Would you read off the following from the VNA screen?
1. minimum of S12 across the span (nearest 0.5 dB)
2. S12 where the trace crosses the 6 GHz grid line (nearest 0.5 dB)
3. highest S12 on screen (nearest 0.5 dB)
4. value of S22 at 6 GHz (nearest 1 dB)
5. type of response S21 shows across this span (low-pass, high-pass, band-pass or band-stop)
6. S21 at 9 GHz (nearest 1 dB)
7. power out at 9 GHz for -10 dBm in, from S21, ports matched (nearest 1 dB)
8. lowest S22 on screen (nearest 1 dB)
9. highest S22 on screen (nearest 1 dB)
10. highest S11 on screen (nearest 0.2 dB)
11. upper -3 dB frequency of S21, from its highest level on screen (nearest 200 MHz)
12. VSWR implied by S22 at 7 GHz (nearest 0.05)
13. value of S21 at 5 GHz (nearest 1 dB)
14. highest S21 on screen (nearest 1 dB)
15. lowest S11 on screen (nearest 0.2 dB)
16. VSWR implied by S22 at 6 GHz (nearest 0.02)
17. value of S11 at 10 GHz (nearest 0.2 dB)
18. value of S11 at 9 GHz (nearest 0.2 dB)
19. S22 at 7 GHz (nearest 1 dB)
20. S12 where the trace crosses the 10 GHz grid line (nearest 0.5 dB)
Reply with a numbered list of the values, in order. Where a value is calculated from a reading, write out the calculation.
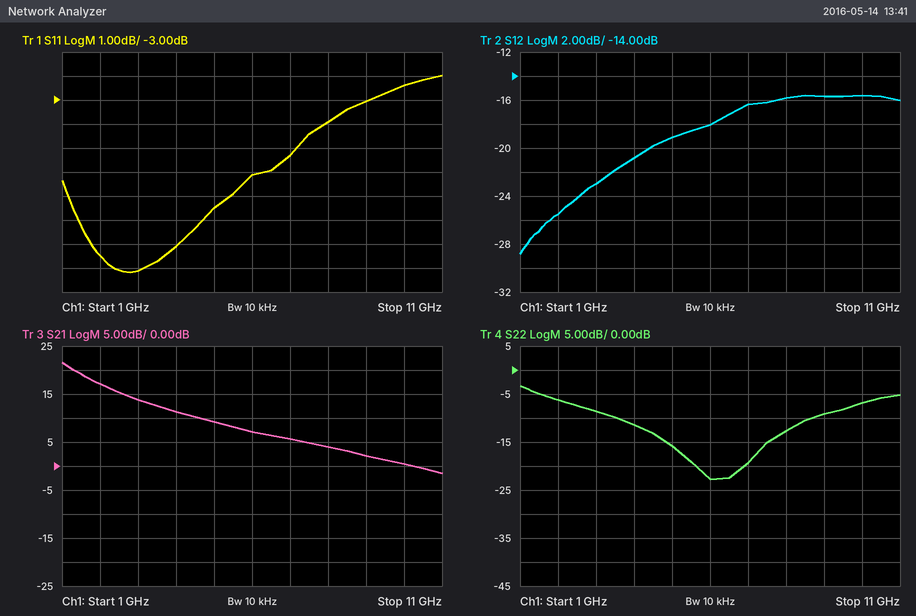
1. -29.0 dB
2. -18.0 dB
3. -15.5 dB
4. -23 dB
5. low-pass
6. 2 dB
7. -10 dBm + (2 dB) = -8 dBm
8. -23 dB
9. -3 dB
10. -2.0 dB
11. 1.6 GHz
12. |Γ| = 10^(-19/20) = 0.1122; VSWR = (1 + 0.1122)/(1 − 0.1122) ≈ 1.25
13. 9 dB
14. 22 dB
15. -10.2 dB
16. |Γ| = 10^(-23/20) = 0.0708; VSWR = (1 + 0.0708)/(1 − 0.0708) ≈ 1.15, so 1.16 to the nearest 0.02
17. -2.4 dB
18. -3.0 dB
19. -19 dB
20. -15.5 dB
